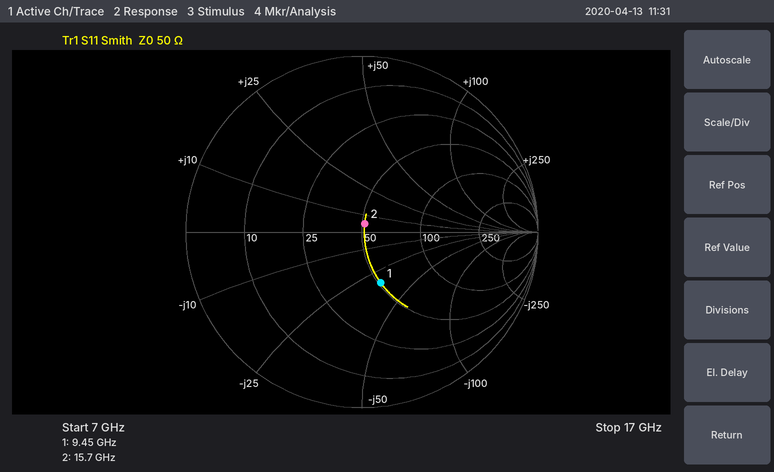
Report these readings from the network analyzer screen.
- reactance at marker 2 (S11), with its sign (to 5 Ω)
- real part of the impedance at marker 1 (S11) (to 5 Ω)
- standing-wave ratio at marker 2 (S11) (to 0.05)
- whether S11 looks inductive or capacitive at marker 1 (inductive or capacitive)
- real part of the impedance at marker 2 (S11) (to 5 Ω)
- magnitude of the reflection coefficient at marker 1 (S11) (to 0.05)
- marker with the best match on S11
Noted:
+5 Ω
50 Ω
1.10
capacitive
50 Ω
0.30
marker 2
